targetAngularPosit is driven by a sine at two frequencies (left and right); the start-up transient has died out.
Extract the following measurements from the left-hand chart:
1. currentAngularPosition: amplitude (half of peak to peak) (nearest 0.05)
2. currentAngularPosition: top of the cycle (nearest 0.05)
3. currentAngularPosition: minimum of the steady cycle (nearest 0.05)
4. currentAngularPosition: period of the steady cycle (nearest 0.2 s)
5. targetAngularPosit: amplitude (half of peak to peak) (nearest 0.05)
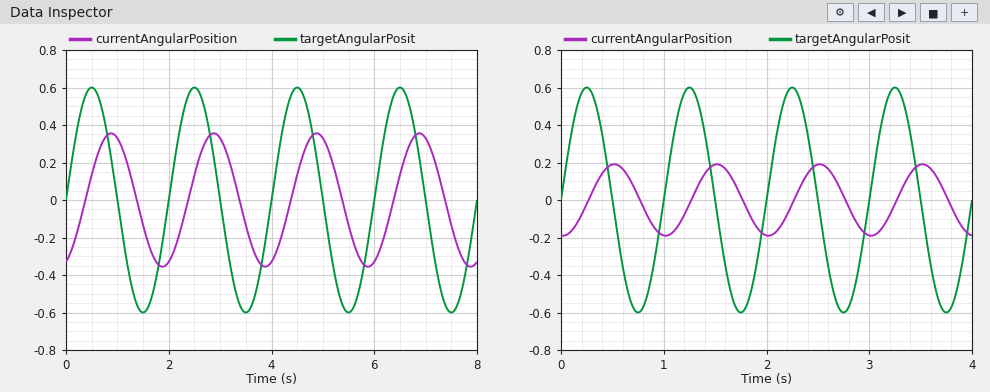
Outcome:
0.35
0.35
-0.35
2.0 s
0.60
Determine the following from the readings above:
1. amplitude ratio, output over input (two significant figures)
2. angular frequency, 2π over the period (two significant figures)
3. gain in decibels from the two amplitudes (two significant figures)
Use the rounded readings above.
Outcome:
0.58
3.1 rad/s
-4.7 dB
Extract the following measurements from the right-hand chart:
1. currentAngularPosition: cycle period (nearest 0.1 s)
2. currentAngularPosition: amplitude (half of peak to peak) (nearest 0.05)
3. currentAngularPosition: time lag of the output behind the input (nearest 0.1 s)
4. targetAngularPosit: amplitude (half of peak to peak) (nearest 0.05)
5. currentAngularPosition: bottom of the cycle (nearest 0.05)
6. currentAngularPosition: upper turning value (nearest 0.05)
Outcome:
1.0 s
0.20
0.3 s
0.60
-0.20
0.20
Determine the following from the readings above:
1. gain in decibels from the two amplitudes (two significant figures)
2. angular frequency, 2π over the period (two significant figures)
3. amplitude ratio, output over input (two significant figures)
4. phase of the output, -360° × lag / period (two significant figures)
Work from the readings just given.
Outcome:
-9.5 dB
6.3 rad/s
0.33
-110°
